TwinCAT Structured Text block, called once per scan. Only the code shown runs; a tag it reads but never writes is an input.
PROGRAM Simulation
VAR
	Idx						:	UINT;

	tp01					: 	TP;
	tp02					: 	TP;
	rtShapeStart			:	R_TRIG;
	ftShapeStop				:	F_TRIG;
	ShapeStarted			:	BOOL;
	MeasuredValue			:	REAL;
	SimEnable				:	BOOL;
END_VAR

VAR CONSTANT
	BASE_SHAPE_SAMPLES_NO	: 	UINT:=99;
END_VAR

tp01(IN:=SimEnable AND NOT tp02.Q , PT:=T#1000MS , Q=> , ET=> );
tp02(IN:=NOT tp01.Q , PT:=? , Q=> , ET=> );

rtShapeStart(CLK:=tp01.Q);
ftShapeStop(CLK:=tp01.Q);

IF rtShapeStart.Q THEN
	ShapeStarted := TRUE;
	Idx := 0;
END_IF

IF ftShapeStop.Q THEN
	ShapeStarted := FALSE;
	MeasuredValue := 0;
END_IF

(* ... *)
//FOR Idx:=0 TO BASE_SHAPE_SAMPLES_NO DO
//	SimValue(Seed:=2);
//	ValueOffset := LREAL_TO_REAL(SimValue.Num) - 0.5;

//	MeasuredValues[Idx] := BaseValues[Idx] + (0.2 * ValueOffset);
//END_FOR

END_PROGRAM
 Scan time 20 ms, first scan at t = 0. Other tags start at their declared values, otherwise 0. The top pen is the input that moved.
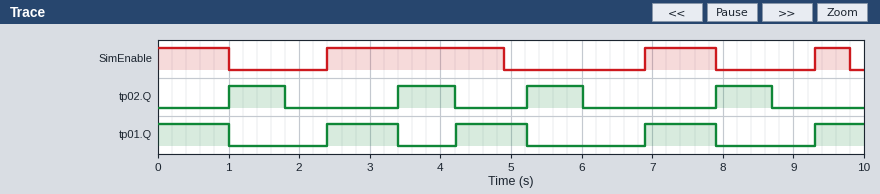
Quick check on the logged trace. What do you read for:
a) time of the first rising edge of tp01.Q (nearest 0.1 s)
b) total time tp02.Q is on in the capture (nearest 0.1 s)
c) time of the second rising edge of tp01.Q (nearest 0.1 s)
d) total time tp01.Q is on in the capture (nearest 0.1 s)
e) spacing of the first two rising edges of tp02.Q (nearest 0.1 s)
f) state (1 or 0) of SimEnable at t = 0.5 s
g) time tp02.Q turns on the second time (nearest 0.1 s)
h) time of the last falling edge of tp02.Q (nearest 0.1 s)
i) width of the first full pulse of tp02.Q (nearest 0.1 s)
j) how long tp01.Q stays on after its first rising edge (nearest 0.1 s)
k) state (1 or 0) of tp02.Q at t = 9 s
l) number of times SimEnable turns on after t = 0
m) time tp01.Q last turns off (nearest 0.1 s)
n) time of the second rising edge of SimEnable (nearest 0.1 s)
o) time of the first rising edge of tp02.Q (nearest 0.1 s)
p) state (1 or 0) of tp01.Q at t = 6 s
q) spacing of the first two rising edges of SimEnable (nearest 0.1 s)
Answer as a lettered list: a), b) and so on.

a) 2.4 s
b) 3.2 s
c) 4.2 s
d) 4.7 s
e) 2.4 s
f) 1
g) 3.4 s
h) 8.7 s
i) 0.8 s
j) 1.0 s
k) 0
l) 3
m) 7.9 s
n) 6.9 s
o) 1.0 s
p) 0
q) 4.5 s
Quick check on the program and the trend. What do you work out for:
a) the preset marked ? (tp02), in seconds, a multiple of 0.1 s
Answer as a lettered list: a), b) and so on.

a) 0.8 s
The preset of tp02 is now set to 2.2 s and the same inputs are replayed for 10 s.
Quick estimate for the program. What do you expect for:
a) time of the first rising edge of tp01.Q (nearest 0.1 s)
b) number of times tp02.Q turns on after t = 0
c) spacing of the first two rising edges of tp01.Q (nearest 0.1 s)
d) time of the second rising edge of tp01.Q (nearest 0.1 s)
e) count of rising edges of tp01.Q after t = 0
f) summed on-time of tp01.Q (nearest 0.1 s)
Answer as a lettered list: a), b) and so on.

a) 3.2 s
b) 3
c) 3.7 s
d) 6.9 s
e) 2
f) 3.0 s
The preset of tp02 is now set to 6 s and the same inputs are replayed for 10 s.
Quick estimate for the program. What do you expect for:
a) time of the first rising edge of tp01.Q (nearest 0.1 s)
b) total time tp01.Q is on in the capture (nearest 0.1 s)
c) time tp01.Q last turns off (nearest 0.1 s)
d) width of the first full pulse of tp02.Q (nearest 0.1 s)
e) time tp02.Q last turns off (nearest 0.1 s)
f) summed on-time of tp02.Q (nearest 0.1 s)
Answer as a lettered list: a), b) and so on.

a) 7.0 s
b) 2.0 s
c) 8.0 s
d) 6.0 s
e) 7.0 s
f) 8.0 s
